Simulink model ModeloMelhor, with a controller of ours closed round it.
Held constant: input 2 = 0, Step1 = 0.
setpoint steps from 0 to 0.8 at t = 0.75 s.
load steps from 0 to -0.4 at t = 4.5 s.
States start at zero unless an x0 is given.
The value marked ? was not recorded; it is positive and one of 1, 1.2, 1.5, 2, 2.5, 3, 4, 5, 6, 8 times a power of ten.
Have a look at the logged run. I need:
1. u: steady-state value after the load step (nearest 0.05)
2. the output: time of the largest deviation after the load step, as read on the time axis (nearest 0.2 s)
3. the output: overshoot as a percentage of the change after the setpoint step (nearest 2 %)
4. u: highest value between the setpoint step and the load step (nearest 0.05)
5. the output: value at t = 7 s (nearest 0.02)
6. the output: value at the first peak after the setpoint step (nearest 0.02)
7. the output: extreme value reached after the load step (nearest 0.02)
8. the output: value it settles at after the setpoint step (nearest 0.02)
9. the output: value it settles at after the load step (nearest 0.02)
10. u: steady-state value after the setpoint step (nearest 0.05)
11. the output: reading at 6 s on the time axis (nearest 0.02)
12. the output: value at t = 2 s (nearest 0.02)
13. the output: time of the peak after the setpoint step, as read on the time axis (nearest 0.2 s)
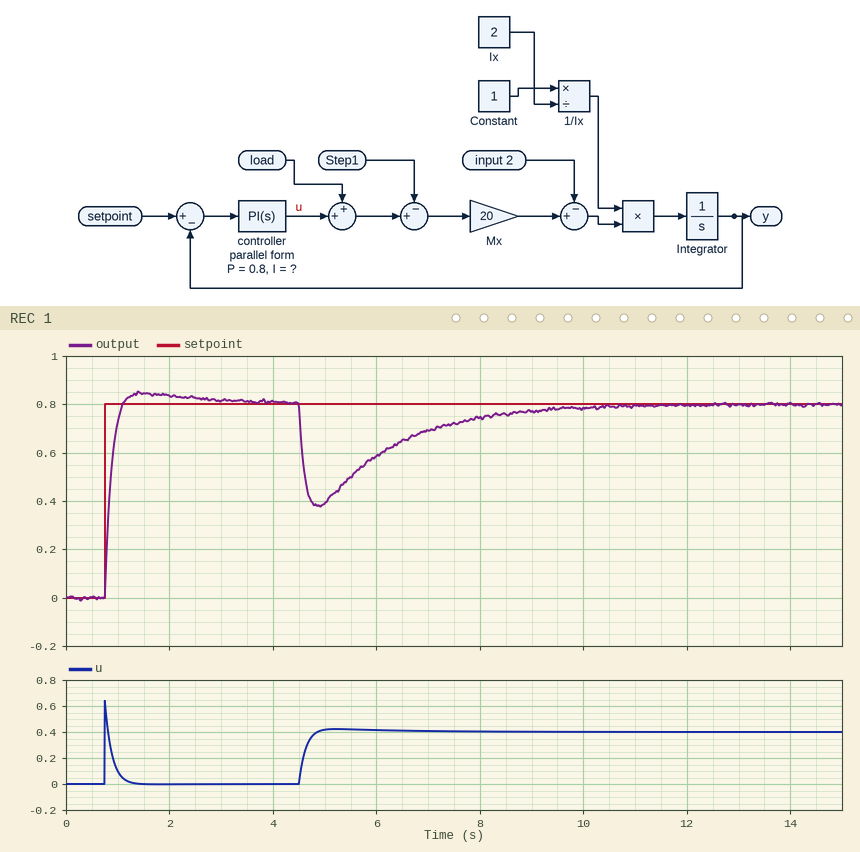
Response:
0.40
4.8 s
6 %
0.65
0.70
0.84
0.38
0.80
0.80
0.00
0.58
0.84
1.4 s
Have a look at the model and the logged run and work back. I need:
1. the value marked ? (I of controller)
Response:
0.5
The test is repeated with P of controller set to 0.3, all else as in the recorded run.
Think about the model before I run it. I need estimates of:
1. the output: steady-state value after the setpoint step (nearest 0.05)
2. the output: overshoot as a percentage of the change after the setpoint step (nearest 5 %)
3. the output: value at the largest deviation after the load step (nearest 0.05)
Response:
0.80
20 %
-0.05
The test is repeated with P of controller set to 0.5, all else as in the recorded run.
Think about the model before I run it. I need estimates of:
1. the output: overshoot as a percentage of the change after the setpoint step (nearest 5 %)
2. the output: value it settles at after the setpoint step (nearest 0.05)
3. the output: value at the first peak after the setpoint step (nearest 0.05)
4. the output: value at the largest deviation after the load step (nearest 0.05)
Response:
10 %
0.80
0.90
0.20
